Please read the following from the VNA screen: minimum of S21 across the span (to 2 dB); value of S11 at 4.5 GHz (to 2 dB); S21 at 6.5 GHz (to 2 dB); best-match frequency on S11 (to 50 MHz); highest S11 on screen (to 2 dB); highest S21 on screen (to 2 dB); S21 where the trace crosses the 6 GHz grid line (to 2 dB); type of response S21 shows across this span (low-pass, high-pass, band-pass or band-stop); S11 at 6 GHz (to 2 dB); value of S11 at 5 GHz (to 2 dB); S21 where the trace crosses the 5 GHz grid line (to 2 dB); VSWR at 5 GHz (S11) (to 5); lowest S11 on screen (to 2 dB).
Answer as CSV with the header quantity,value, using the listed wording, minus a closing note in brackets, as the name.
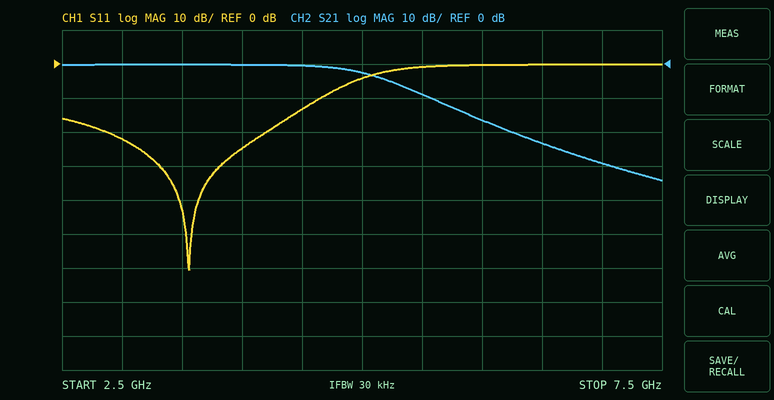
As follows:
quantity,value
minimum of S21 across the span,-34 dB
value of S11 at 4.5 GHz,-14 dB
S21 at 6.5 GHz,-24 dB
best-match frequency on S11,3.55 GHz
highest S11 on screen,0 dB
highest S21 on screen,0 dB
S21 where the trace crosses the 6 GHz grid line,-16 dB
type of response S21 shows across this span,low-pass
S11 at 6 GHz,0 dB
value of S11 at 5 GHz,-4 dB
S21 where the trace crosses the 5 GHz grid line,-2 dB
VSWR at 5 GHz (S11),5
lowest S11 on screen,-60 dB
